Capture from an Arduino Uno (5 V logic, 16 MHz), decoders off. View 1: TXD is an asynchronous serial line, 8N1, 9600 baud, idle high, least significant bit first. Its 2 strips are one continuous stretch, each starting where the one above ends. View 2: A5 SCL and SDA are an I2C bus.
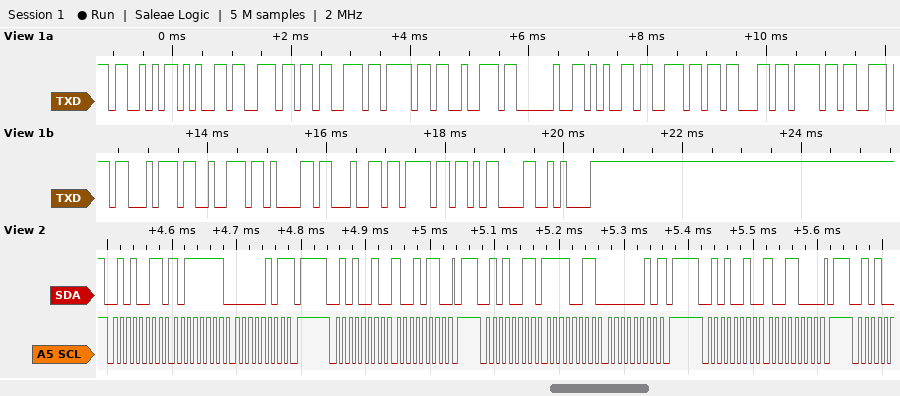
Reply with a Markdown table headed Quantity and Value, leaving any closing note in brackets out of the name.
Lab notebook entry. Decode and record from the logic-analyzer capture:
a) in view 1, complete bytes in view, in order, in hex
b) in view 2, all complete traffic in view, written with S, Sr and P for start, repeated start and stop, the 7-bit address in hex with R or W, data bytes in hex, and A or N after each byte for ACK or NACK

| Quantity | Value |
|---|---|
| in view 1, complete bytes in view, in order, in hex | 53 65 6E 73 6F 72 20 65 6E 63 6F 6E 74 72 61 64 6F 0D 0A |
| in view 2, all complete traffic in view, written with S, Sr and P for start, repeated start and stop, the 7-bit address in hex with R or W, data bytes in hex, and A or N after each byte for ACK or NACK | S 29R A BF A 05 N P S 29W A 96 A P S 29R A F3 A 02 N P S 29W A 98 A P |
